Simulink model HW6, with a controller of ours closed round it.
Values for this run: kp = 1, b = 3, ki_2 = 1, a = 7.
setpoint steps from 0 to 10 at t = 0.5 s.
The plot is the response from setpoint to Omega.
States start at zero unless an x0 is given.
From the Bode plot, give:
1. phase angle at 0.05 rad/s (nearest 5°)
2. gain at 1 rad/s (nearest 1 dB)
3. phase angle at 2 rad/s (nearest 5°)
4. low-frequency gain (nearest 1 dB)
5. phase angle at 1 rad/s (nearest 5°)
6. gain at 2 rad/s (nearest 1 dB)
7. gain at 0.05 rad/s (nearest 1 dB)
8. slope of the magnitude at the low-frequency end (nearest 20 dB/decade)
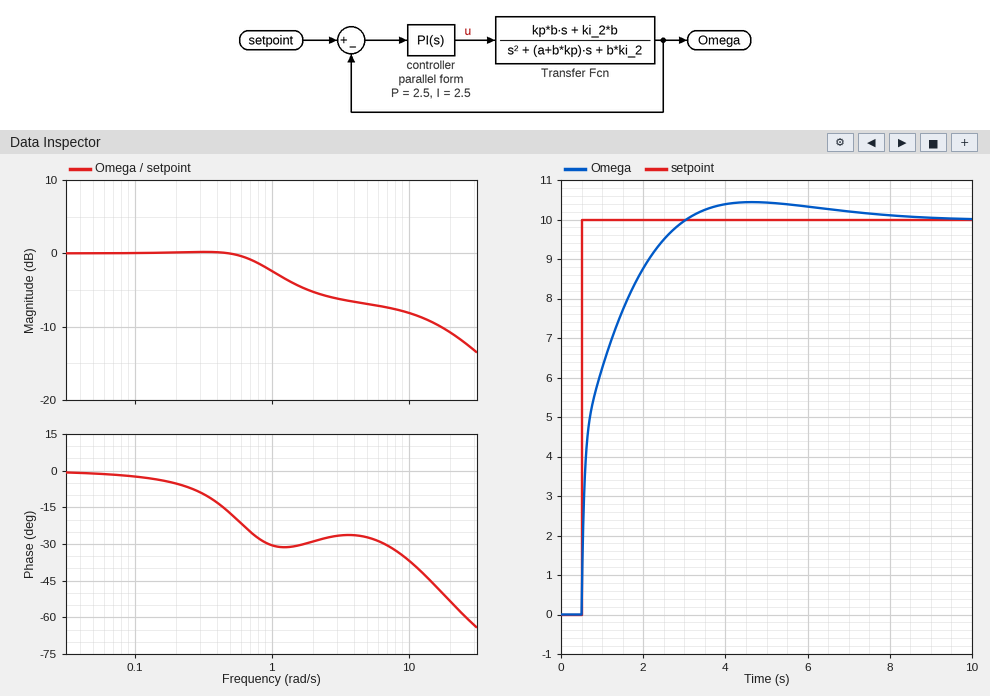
0°
-2 dB
-30°
0 dB
-30°
-5 dB
0 dB
0 dB/decade
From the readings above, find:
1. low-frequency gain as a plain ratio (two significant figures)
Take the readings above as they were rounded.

1.0
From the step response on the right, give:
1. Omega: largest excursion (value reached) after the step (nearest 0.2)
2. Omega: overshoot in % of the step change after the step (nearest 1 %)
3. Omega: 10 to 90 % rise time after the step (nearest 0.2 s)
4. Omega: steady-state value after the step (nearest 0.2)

10.4
4 %
1.6 s
10.0
